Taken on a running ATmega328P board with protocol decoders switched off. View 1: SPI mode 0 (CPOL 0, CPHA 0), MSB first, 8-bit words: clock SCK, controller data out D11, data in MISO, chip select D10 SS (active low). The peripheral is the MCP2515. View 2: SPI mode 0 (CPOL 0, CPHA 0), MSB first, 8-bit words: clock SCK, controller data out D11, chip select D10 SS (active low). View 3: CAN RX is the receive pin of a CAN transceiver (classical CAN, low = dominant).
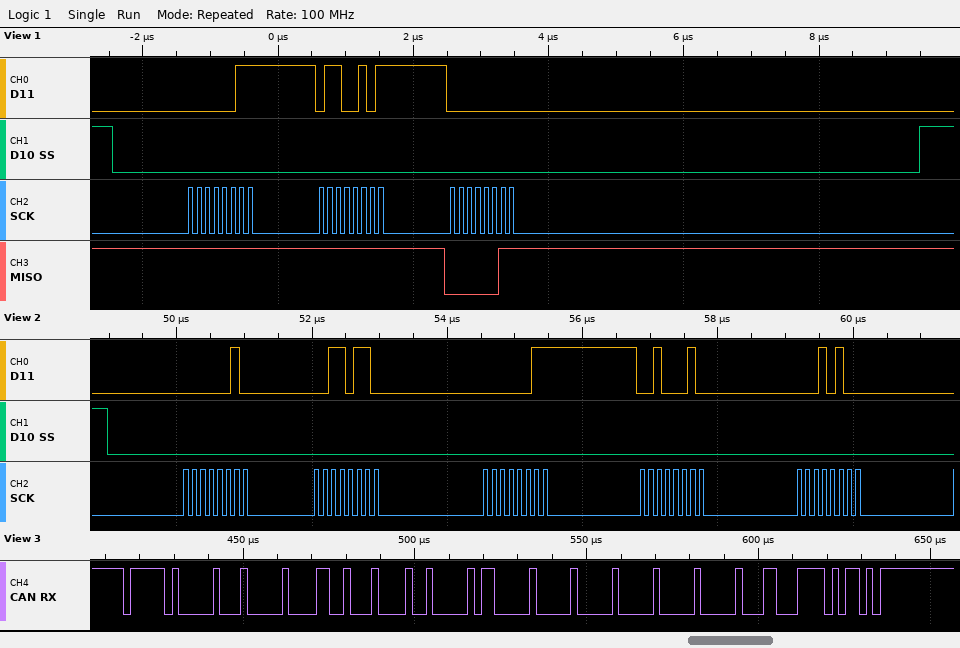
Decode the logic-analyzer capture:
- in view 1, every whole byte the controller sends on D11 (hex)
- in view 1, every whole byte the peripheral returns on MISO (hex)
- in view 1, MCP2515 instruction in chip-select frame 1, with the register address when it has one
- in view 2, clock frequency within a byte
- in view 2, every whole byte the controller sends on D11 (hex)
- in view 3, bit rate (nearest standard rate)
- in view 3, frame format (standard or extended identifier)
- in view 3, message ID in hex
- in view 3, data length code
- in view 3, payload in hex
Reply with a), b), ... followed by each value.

a) 03 65 00
b) FF FF 03
c) READ 0x65
d) 8 MHz
e) 0x02 0x36 0x03 0x22 0x14
f) 500 kbit/s
g) standard
h) 0x7E0
i) 8
j) 03 22 12 06 00 00 00 00
